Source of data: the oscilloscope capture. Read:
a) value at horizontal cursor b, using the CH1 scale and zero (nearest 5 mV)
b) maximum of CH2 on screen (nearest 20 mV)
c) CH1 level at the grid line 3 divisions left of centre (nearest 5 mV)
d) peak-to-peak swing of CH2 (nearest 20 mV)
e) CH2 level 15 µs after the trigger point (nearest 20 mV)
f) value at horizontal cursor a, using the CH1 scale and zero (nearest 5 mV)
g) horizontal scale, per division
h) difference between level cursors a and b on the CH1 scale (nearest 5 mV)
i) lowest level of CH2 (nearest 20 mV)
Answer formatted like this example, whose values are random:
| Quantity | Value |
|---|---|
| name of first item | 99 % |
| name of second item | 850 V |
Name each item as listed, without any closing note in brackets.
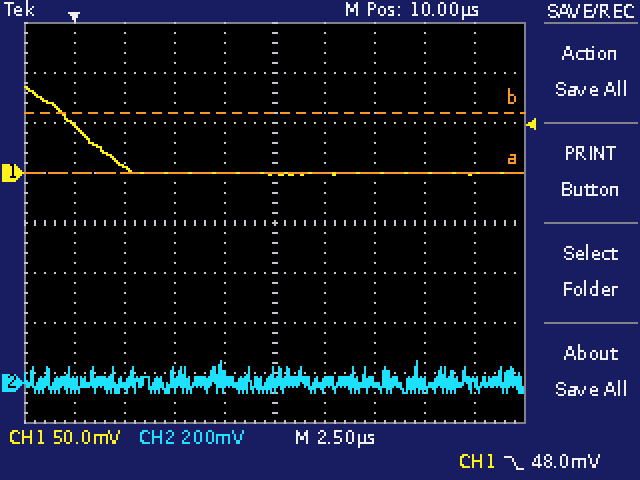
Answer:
| Quantity | Value |
|---|---|
| value at horizontal cursor b, using the CH1 scale and zero | 60 mV |
| maximum of CH2 on screen | 80 mV |
| CH1 level at the grid line 3 divisions left of centre | 5 mV |
| peak-to-peak swing of CH2 | 120 mV |
| CH2 level 15 µs after the trigger point | 0 mV |
| value at horizontal cursor a, using the CH1 scale and zero | 0 mV |
| horizontal scale, per division | 2.5 µs |
| difference between level cursors a and b on the CH1 scale | 60 mV |
| lowest level of CH2 | -40 mV |
